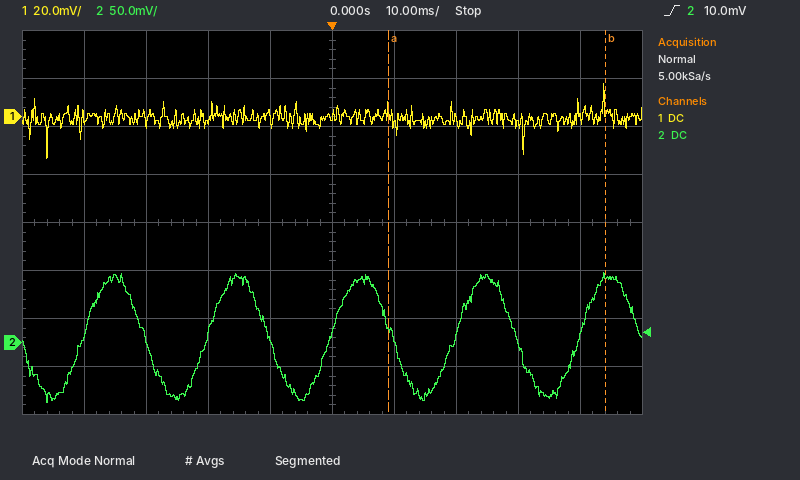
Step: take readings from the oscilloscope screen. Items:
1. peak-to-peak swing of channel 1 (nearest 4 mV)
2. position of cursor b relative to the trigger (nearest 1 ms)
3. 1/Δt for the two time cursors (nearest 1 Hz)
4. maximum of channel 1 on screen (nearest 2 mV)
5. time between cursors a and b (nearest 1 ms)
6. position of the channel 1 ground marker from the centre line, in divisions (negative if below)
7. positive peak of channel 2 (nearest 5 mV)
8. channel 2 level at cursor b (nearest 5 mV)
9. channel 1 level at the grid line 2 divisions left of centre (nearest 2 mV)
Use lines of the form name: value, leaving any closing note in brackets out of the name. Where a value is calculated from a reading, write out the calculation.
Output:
peak-to-peak swing of channel 1: 32 mV
position of cursor b relative to the trigger: +44 ms
1/Δt for the two time cursors: 1 / 35 ms ≈ 29 Hz
maximum of channel 1 on screen: 14 mV
time between cursors a and b: 35 ms
position of the channel 1 ground marker from the centre line, in divisions: +2.2 div
positive peak of channel 2: 75 mV
channel 2 level at cursor b: 70 mV
channel 1 level at the grid line 2 divisions left of centre: -2 mV
